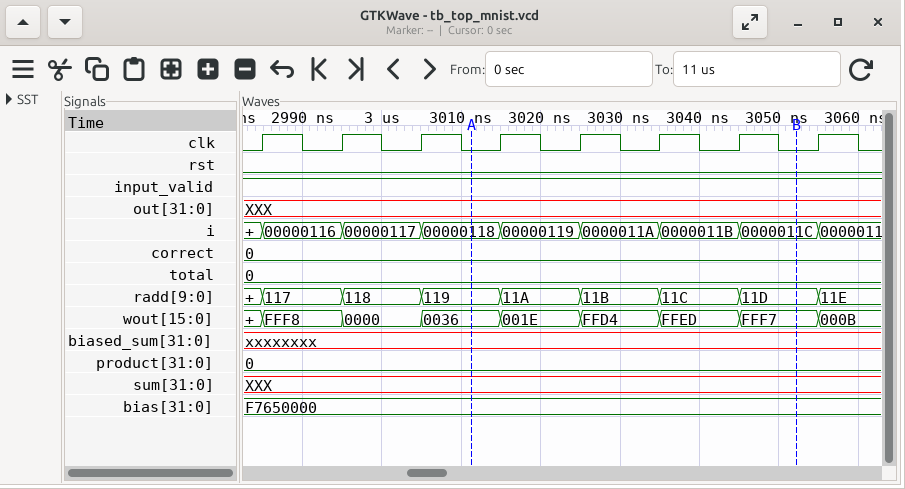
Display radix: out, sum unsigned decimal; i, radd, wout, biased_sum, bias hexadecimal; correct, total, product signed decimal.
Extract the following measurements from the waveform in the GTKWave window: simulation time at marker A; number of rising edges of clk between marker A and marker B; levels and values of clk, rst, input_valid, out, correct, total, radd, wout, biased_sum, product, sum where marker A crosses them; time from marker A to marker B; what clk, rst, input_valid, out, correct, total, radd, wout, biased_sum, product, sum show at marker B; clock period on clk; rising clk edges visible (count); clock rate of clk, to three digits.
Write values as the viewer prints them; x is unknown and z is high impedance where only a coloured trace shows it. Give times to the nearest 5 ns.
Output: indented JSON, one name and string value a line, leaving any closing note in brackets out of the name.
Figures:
{
  "simulation time at marker A": "3010 ns",
  "number of rising edges of clk between marker A and marker B": "4",
  "levels and values of clk, rst, input_valid, out, correct, total, radd, wout, biased_sum, product, sum where marker A crosses them": "clk=0, rst=0, input_valid=1, out=XXX, correct=0, total=0, radd=119, wout=0036, biased_sum=xxxxxxxx, product=0, sum=XXX",
  "time from marker A to marker B": "40 ns",
  "what clk, rst, input_valid, out, correct, total, radd, wout, biased_sum, product, sum show at marker B": "clk=0, rst=0, input_valid=1, out=XXX, correct=0, total=0, radd=11D, wout=FFF7, biased_sum=xxxxxxxx, product=0, sum=XXX",
  "clock period on clk": "10 ns",
  "rising clk edges visible": "8",
  "clock rate of clk, to three digits": "100 MHz"
}
